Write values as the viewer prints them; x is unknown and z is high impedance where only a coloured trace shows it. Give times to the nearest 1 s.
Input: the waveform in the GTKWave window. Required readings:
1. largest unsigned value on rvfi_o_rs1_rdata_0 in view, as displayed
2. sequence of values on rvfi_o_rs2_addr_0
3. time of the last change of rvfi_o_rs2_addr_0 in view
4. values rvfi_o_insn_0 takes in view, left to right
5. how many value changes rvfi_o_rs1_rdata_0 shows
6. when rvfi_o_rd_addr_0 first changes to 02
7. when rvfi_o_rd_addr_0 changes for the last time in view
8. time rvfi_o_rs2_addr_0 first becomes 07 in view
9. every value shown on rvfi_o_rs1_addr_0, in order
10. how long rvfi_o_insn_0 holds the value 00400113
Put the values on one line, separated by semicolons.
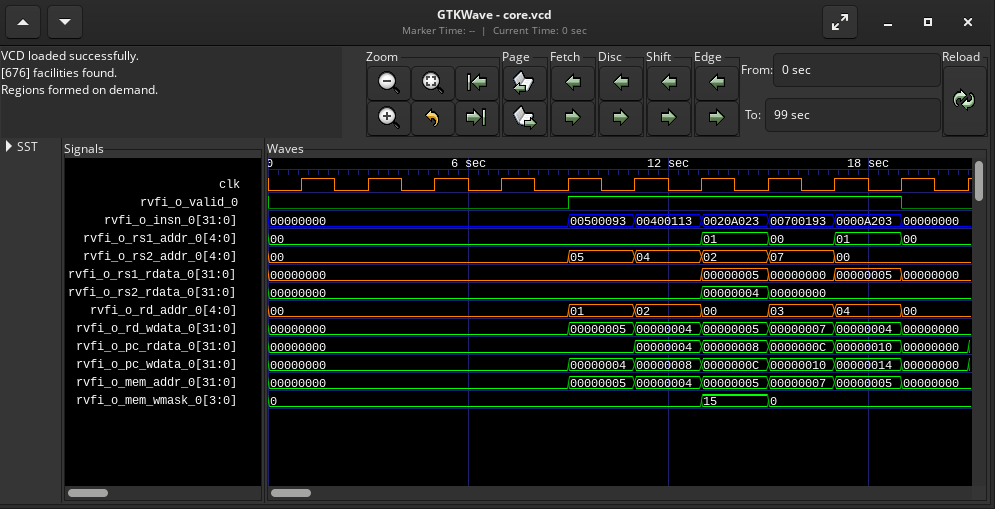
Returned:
00000005; 00, 05, 04, 02, 07, 00; 17 s; 00000000, 00500093, 00400113, 0020A023, 00700193, 0000A203, 00000000; 4; 11 s; 19 s; 15 s; 00, 01, 00, 01, 00; 2 s
